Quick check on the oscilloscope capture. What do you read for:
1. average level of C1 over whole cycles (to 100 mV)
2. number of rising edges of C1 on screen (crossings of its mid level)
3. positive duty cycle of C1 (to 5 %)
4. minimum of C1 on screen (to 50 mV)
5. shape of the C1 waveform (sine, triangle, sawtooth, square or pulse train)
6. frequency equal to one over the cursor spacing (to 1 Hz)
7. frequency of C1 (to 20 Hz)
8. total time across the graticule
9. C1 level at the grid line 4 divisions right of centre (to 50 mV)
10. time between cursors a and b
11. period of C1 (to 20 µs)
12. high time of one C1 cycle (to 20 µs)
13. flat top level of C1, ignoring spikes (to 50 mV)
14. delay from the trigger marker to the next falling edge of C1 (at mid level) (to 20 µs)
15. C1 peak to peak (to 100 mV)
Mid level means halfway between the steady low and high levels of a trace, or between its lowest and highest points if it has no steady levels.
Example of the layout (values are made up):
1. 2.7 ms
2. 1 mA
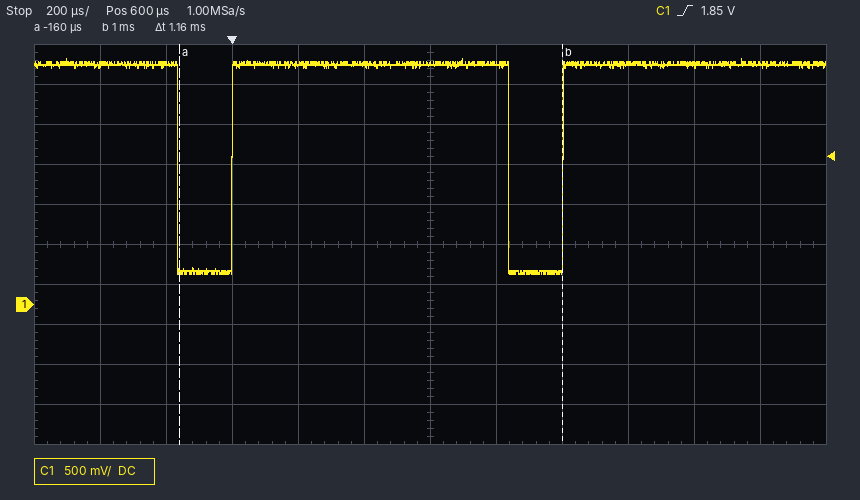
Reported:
1. 2.6 V
2. 2
3. 85 %
4. 400 mV
5. pulse train
6. 862 Hz
7. 1.00 kHz
8. 2.4 ms
9. 3.00 V
10. 1.16 ms
11. 1.00 ms
12. 840 µs
13. 3.00 V
14. 840 µs
15. 2.70 V
